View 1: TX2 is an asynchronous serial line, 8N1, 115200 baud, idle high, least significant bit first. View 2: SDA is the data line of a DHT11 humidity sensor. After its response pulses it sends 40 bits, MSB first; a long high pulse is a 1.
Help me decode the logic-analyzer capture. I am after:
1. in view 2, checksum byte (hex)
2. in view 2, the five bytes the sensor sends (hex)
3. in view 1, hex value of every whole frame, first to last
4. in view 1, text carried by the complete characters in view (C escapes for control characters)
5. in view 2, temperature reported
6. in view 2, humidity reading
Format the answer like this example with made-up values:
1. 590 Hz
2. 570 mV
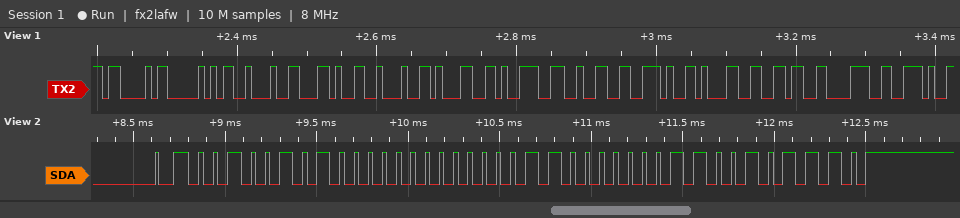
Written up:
1. 0x2E
2. 25 00 06 03 2E
3. 43 50 22 2C 22 31 39 32 2E 31 36 38 2E
4. "CP\",\"192.168."
5. 6.3 °C
6. 37 %
